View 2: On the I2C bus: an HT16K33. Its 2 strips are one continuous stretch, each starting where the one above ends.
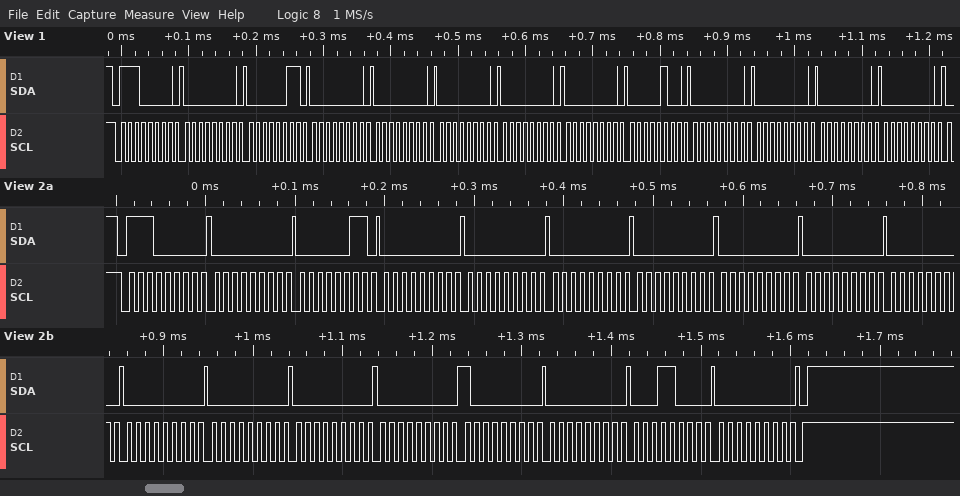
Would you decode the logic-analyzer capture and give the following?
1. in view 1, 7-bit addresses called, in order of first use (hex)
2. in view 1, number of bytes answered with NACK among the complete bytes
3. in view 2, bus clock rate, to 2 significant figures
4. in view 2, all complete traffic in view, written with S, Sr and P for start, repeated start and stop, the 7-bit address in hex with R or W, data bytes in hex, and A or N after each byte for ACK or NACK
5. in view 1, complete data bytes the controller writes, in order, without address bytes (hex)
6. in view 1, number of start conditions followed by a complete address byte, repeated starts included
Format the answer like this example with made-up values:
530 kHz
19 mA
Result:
0x70
0
100 kHz
S 70W A 00 A 03 A 00 A 00 A 00 A 00 A 00 A 00 A 00 A 00 A 00 A 00 A 00 A 80 A 00 A 18 A 00 A P
00 03 00 00 00 00 00 04 00 00 00 00
1
